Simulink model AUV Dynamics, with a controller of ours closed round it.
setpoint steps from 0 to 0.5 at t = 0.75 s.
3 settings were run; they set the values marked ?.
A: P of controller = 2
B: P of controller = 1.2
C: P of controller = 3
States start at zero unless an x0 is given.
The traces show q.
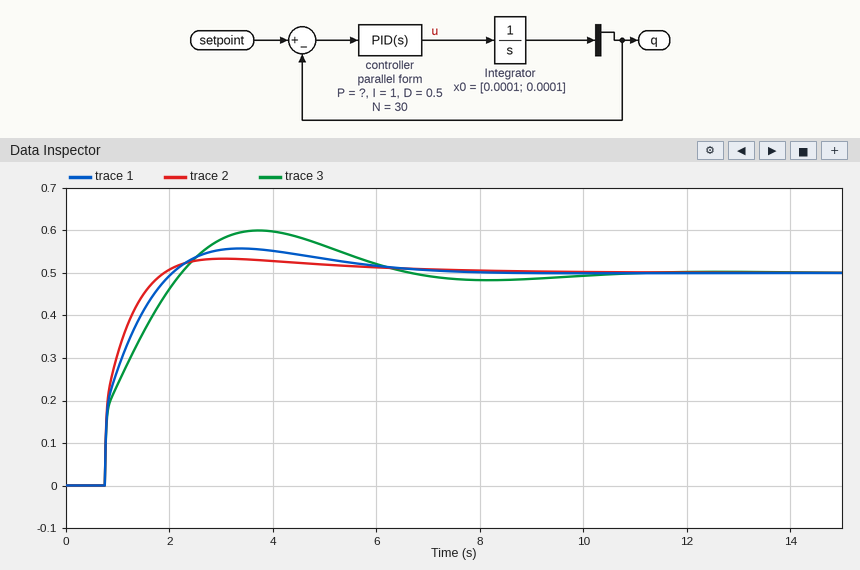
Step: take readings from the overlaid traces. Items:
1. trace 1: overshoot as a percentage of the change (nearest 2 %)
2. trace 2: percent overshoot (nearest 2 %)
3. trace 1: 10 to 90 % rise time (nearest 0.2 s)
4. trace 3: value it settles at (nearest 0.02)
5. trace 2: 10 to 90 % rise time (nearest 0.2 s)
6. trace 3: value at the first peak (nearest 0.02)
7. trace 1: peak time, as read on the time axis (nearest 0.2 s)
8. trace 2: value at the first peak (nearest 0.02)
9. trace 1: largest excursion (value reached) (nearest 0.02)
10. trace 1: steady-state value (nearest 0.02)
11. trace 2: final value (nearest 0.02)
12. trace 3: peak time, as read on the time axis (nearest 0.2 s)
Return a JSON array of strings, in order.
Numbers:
["12 %", "6 %", "1.0 s", "0.50", "0.8 s", "0.60", "3.4 s", "0.54", "0.56", "0.50", "0.50", "3.8 s"]
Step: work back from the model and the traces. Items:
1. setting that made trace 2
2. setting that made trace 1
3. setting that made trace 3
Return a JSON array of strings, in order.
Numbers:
["C", "A", "B"]
